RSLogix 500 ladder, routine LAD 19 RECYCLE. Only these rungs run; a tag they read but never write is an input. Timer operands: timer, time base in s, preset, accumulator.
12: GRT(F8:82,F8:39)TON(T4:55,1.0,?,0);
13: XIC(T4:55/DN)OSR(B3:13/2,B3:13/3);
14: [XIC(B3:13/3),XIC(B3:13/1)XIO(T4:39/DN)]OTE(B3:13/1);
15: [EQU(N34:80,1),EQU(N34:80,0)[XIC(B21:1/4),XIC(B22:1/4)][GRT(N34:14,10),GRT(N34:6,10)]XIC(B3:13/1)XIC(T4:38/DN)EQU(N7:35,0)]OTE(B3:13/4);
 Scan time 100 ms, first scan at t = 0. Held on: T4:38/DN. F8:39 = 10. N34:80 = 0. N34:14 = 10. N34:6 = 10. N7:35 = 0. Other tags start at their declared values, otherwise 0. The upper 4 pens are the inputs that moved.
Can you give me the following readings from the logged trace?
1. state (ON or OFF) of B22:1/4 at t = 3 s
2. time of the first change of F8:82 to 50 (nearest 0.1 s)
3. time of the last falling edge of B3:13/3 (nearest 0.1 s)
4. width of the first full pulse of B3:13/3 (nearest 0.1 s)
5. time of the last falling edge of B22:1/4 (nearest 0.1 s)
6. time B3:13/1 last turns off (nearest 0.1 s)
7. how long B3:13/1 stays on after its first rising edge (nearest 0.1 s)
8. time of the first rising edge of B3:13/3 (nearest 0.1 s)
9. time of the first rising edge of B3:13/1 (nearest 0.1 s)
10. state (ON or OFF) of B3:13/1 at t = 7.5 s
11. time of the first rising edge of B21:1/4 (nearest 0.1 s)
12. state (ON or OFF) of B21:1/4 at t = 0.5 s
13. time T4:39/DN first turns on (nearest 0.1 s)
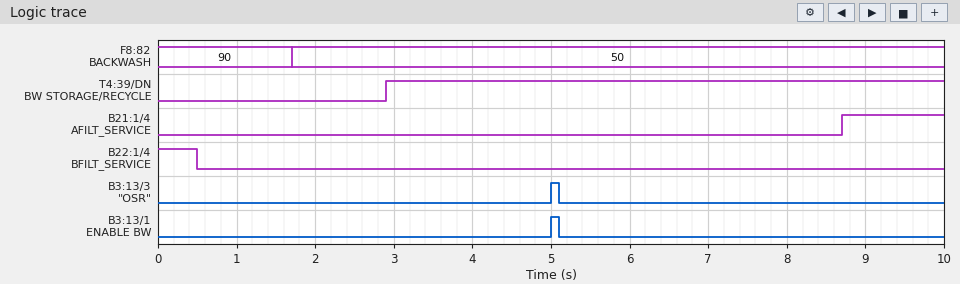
OFF
1.7 s
5.1 s
0.1 s
0.5 s
5.1 s
0.1 s
5.0 s
5.0 s
OFF
8.7 s
OFF
2.9 s
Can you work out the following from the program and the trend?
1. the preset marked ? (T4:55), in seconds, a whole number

5 s
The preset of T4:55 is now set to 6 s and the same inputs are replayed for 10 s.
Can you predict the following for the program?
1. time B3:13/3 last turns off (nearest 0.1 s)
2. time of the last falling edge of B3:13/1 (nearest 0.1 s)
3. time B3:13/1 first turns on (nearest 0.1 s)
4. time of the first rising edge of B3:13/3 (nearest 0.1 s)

6.1 s
6.1 s
6.0 s
6.0 s
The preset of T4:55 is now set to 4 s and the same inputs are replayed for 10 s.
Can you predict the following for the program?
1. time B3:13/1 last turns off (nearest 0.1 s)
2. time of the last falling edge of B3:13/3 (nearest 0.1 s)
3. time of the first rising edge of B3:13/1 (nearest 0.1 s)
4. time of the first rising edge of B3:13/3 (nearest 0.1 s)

4.1 s
4.1 s
4.0 s
4.0 s
